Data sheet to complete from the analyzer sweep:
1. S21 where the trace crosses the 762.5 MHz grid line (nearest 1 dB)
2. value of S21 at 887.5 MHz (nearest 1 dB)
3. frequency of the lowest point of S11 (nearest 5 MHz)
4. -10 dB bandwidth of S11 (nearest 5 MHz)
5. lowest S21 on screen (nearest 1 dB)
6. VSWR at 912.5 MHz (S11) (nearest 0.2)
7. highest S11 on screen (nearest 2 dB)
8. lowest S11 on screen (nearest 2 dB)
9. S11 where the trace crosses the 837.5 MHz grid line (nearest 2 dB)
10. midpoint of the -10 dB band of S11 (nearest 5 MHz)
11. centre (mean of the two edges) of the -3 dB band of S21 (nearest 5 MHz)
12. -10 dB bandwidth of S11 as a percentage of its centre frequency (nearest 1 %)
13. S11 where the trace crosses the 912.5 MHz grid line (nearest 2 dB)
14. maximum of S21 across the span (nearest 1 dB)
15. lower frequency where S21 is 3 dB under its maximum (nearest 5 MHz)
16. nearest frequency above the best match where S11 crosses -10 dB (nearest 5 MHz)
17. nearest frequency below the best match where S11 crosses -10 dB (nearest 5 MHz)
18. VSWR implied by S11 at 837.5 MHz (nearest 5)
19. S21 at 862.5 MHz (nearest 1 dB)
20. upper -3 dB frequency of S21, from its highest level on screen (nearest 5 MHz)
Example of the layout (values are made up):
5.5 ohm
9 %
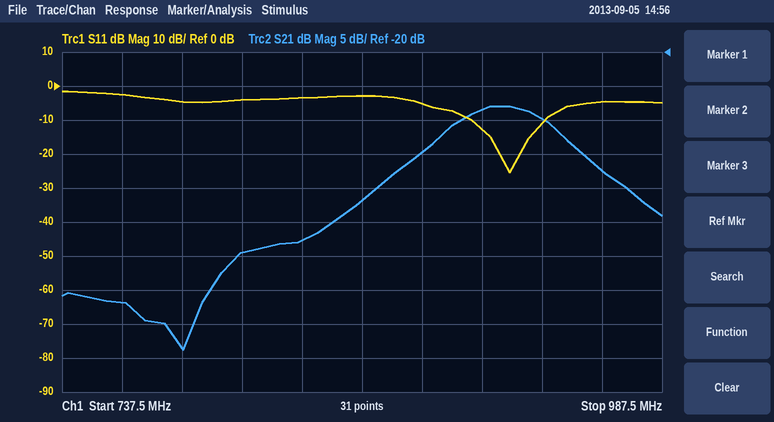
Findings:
-57 dB
-35 dB
925 MHz
30 MHz
-64 dB
1.6
-2 dB
-26 dB
-4 dB
925 MHz
920 MHz
3 %
-12 dB
-28 dB
900 MHz
940 MHz
910 MHz
5
-42 dB
940 MHz
